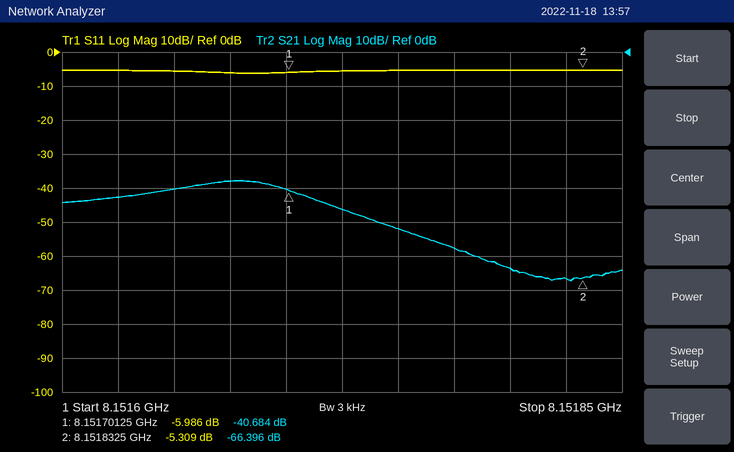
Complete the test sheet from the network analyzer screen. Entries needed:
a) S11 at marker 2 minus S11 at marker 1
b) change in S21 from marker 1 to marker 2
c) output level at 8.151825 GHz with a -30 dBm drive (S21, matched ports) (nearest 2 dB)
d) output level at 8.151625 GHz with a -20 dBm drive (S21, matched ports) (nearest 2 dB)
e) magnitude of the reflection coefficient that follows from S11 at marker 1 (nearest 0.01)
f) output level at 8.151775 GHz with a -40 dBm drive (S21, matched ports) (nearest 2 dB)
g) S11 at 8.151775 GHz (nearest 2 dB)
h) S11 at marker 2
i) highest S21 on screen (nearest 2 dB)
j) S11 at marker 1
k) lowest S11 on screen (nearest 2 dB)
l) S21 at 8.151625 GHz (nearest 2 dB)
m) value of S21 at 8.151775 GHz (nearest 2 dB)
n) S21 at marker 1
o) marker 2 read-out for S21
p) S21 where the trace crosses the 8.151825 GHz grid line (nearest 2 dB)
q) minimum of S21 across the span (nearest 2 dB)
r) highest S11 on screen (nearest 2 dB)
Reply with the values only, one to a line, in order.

0.677 dB
-25.712 dB
-96 dBm
-62 dBm
0.50
-98 dBm
-6 dB
-5.309 dB
-38 dB
-5.986 dB
-6 dB
-42 dB
-58 dB
-40.684 dB
-66.396 dB
-66 dB
-68 dB
-6 dB
